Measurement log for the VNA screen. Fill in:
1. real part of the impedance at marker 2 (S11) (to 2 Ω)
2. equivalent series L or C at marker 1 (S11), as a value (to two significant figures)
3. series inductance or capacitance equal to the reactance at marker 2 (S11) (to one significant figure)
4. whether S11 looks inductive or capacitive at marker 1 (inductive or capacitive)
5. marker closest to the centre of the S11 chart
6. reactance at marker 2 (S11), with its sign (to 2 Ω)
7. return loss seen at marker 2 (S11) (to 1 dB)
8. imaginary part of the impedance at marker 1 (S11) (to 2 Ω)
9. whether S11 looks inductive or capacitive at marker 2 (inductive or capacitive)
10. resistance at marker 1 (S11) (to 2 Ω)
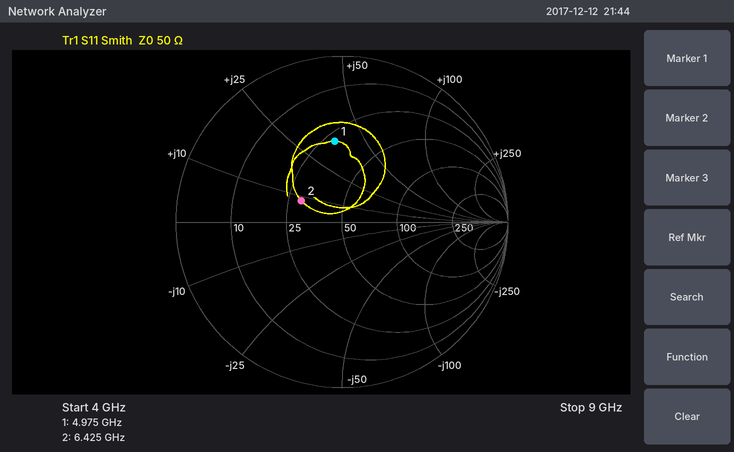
30 Ω
1.2 nH
200 pH
inductive
marker 2
+8 Ω
11 dB
+36 Ω
inductive
28 Ω
